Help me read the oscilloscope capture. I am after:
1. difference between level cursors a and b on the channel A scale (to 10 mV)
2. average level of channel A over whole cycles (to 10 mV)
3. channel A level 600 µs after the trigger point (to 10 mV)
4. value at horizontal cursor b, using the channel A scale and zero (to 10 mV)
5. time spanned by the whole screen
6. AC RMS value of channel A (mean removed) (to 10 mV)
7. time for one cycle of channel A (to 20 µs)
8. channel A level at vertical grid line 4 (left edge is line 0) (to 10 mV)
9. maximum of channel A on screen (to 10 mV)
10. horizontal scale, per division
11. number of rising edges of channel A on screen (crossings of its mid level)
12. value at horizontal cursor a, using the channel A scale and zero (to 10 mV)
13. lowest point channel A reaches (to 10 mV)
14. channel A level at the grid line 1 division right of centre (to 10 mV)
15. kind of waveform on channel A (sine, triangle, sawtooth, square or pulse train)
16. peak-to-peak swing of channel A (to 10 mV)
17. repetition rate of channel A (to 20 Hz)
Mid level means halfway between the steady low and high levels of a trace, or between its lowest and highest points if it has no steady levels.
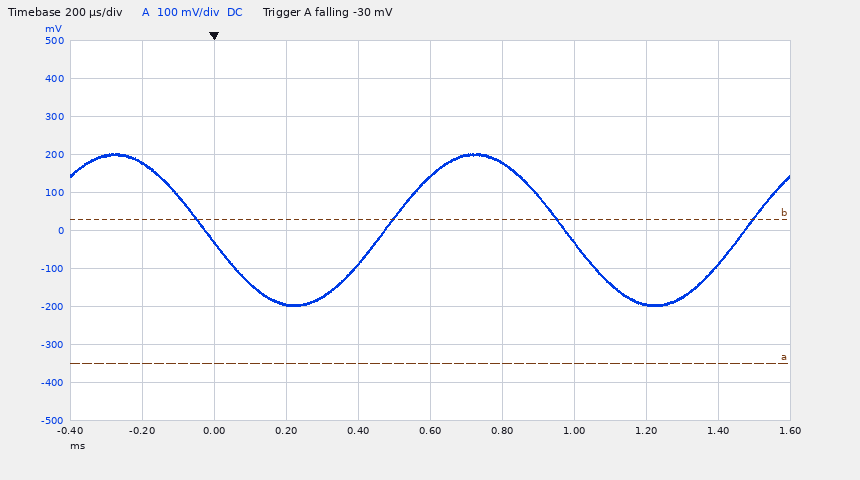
380 mV
0 mV
140 mV
30 mV
2 ms
140 mV
1.00 ms
-90 mV
200 mV
200 µs
2
-350 mV
-200 mV
180 mV
sine
400 mV
1.00 kHz
